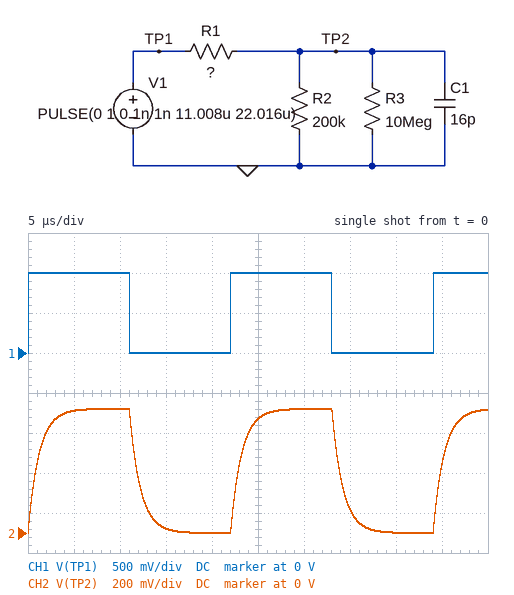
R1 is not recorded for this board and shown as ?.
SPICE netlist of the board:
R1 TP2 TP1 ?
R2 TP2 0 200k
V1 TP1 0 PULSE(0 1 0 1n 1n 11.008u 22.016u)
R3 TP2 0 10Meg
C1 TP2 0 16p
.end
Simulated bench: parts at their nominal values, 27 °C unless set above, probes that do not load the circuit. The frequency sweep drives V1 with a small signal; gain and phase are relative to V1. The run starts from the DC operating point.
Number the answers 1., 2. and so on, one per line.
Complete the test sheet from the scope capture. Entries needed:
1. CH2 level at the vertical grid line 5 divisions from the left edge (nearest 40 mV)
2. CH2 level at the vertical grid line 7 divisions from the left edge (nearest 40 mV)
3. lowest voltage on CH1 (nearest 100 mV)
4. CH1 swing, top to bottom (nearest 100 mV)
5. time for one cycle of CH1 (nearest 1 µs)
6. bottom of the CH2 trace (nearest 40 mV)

1. 560 mV
2. 120 mV
3. 0 V
4. 1.0 V
5. 22 µs
6. 0 V
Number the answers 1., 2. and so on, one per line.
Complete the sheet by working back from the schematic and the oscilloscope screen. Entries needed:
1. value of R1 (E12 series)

1. 120 kΩ
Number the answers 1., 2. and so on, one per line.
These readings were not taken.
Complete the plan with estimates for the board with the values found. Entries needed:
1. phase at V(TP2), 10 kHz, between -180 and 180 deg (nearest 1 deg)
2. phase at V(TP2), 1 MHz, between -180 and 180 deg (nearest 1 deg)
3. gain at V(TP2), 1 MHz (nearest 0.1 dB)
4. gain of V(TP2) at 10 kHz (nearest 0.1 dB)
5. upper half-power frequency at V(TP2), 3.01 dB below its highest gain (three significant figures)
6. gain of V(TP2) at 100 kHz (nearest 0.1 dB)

1. -4 deg
2. -82 deg
3. -21.7 dB
4. -4.2 dB
5. 134 kHz
6. -6.1 dB
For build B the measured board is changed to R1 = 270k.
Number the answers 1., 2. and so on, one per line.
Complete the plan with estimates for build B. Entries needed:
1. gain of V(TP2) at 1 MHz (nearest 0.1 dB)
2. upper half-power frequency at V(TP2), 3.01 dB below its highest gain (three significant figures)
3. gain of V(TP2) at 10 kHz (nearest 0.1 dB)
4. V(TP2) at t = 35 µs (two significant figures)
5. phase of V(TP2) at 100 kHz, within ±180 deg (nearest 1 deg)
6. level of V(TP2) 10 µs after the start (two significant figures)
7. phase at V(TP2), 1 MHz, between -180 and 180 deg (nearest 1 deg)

1. -28.7 dB
2. 87.6 kHz
3. -7.6 dB
4. 140 mV
5. -49 deg
6. 420 mV
7. -85 deg
